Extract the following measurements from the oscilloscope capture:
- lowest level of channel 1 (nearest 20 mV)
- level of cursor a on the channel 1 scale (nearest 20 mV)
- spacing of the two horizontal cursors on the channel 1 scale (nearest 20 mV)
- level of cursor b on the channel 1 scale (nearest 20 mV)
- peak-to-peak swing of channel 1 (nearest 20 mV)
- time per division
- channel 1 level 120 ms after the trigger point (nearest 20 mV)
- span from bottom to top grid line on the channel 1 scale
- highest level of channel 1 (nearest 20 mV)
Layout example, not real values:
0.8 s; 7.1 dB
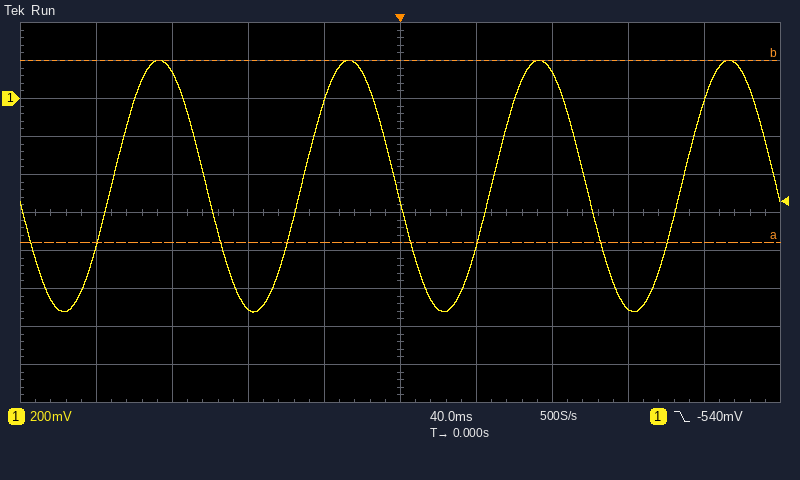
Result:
-1.12 V; -760 mV; 960 mV; 200 mV; 1.32 V; 40 ms; -1.10 V; 2 V; 200 mV
